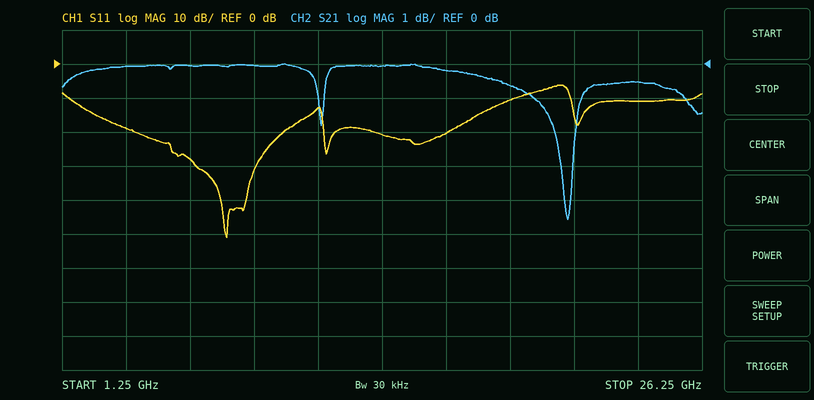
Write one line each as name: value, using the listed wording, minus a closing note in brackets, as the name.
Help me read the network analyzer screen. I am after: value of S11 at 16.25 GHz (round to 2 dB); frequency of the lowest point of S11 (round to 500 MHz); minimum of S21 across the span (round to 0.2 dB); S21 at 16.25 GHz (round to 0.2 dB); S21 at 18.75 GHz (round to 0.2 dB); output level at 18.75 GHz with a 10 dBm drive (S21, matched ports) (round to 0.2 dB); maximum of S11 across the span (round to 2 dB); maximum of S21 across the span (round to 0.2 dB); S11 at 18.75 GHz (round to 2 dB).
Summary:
value of S11 at 16.25 GHz: -20 dB
frequency of the lowest point of S11: 7.5 GHz
minimum of S21 across the span: -4.6 dB
S21 at 16.25 GHz: -0.2 dB
S21 at 18.75 GHz: -0.6 dB
output level at 18.75 GHz with a 10 dBm drive (S21, matched ports): 9.4 dBm
maximum of S11 across the span: -6 dB
maximum of S21 across the span: 0.0 dB
S11 at 18.75 GHz: -10 dB
